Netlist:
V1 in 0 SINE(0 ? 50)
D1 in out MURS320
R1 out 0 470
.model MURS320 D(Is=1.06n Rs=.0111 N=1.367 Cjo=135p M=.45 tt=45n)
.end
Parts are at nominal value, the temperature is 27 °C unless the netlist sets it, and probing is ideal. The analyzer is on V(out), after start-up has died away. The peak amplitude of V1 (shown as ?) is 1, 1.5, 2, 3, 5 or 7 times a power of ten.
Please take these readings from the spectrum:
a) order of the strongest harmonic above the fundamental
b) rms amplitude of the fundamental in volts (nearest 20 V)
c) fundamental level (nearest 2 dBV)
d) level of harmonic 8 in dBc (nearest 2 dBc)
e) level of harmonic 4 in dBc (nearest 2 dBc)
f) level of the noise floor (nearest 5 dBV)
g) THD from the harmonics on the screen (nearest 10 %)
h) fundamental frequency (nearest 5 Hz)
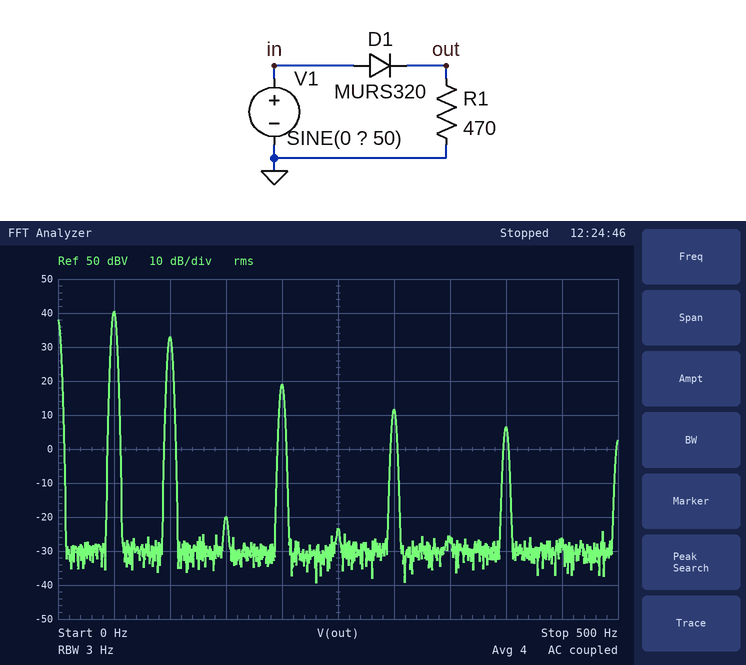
2
100 V
40 dBV
-34 dBc
-22 dBc
-30 dBV
40 %
50 Hz
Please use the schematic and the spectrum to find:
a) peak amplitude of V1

300 V
